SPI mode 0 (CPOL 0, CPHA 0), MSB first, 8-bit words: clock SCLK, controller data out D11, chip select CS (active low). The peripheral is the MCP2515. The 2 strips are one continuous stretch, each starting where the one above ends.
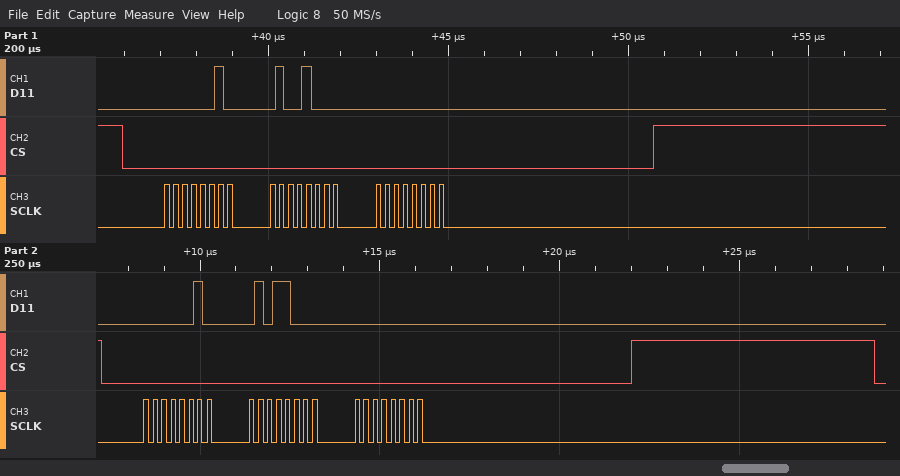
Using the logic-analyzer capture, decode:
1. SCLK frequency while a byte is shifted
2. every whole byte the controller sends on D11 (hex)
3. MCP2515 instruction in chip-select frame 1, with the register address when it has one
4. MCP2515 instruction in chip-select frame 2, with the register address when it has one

4 MHz
02 48 00 02 58 00
WRITE 0x48
WRITE 0x58
